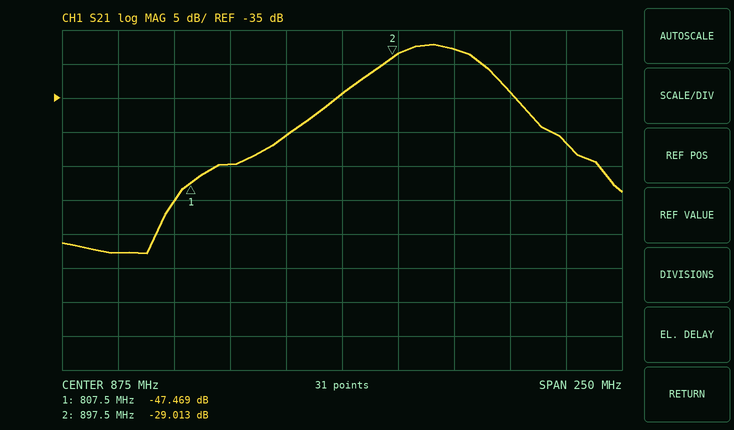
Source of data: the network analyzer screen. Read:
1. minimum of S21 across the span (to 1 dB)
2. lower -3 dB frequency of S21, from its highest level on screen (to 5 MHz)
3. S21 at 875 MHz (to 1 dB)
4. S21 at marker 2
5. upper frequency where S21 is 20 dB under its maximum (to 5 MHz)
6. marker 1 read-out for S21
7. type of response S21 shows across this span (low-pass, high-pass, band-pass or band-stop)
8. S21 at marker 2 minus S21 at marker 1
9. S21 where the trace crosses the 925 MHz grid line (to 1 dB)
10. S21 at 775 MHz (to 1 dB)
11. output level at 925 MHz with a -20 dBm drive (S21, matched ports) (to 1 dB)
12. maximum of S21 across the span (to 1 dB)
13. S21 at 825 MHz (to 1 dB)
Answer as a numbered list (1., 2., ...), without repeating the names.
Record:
1. -58 dB
2. 895 MHz
3. -34 dB
4. -29.013 dB
5. 995 MHz
6. -47.469 dB
7. band-pass
8. 18.456 dB
9. -28 dB
10. -58 dB
11. -48 dBm
12. -27 dB
13. -45 dB
